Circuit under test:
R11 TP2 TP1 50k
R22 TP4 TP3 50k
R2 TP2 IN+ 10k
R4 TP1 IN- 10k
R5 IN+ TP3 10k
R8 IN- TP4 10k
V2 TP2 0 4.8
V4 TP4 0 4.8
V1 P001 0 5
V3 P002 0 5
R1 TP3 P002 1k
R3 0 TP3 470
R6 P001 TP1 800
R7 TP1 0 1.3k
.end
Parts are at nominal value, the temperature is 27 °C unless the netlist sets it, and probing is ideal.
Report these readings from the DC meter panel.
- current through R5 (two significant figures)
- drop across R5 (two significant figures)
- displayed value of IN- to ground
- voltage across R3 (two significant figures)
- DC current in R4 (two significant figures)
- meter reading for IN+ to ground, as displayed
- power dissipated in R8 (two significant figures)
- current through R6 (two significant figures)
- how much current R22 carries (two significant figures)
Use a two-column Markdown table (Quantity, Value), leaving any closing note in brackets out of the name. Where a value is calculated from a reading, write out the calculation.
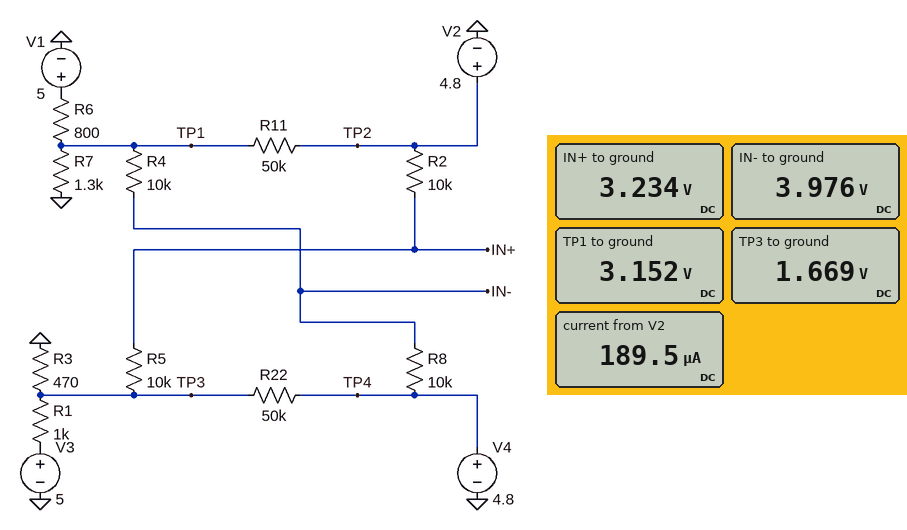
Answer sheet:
| Quantity | Value |
|---|---|
| current through R5 | (3.234 V - 1.669 V) / 10 kΩ = 160 µA |
| drop across R5 | 3.234 V - 1.669 V = 1.6 V |
| displayed value of IN- to ground | 3.976 V |
| voltage across R3 | 1.669 V = 1.7 V |
| DC current in R4 | (3.976 V - 3.152 V) / 10 kΩ = 82 µA |
| meter reading for IN+ to ground, as displayed | 3.234 V |
| power dissipated in R8 | (4.8 V - 3.976 V)^2 / 10 kΩ = 68 µW |
| current through R6 | (5 V - 3.152 V) / 800 Ω = 2.3 mA |
| how much current R22 carries | (4.8 V - 1.669 V) / 50 kΩ = 63 µA |
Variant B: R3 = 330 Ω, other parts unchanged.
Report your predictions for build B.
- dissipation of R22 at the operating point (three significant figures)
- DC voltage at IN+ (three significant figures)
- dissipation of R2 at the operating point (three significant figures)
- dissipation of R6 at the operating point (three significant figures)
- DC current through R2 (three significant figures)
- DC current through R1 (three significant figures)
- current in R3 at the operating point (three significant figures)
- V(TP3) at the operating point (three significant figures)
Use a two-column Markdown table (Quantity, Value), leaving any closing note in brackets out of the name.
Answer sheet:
| Quantity | Value |
|---|---|
| dissipation of R22 at the operating point | 245 µW |
| DC voltage at IN+ | 3.05 V |
| dissipation of R2 at the operating point | 306 µW |
| dissipation of R6 at the operating point | 4.27 mW |
| DC current through R2 | 175 µA |
| DC current through R1 | 3.70 mA |
| current in R3 at the operating point | 3.94 mA |
| V(TP3) at the operating point | 1.30 V |
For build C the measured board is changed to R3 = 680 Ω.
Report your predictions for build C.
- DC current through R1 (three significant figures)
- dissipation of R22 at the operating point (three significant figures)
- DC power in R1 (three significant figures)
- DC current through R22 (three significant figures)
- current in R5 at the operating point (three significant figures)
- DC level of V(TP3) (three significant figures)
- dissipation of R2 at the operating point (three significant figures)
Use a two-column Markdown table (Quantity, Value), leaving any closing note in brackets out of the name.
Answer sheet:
| Quantity | Value |
|---|---|
| DC current through R1 | 2.90 mA |
| dissipation of R22 at the operating point | 146 µW |
| DC power in R1 | 8.41 mW |
| DC current through R22 | 54.0 µA |
| current in R5 at the operating point | 135 µA |
| DC level of V(TP3) | 2.10 V |
| dissipation of R2 at the operating point | 182 µW |
